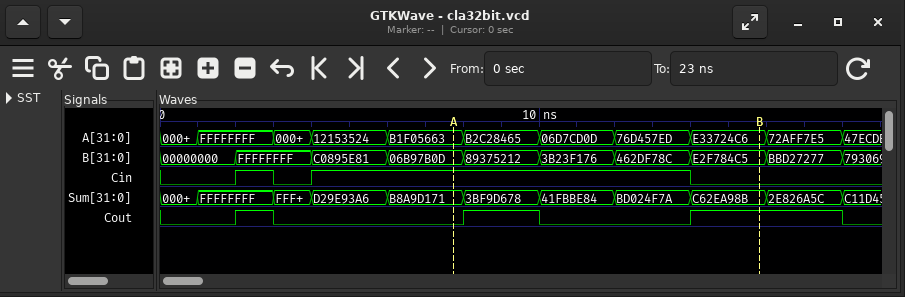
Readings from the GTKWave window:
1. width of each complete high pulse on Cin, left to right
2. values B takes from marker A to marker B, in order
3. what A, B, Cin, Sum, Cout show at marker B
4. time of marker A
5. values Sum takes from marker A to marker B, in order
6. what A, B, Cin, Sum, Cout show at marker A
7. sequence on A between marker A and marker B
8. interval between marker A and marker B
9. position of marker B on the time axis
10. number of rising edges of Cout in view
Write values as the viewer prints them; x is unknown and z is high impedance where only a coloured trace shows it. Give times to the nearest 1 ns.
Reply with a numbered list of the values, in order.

1. 1 ns, 10 ns
2. 06B97B0D, 89375212, 3B23F176, 462DF78C, E2F784C5
3. A=E33724C6, B=E2F784C5, Cin=0, Sum=C62EA98B, Cout=1
4. 8 ns
5. B8A9D171, 3BF9D678, 41FBBE84, BD024F7A, C62EA98B
6. A=B1F05663, B=06B97B0D, Cin=1, Sum=B8A9D171, Cout=0
7. B1F05663, B2C28465, 06D7CD0D, 76D457ED, E33724C6
8. 8 ns
9. 16 ns
10. 3
